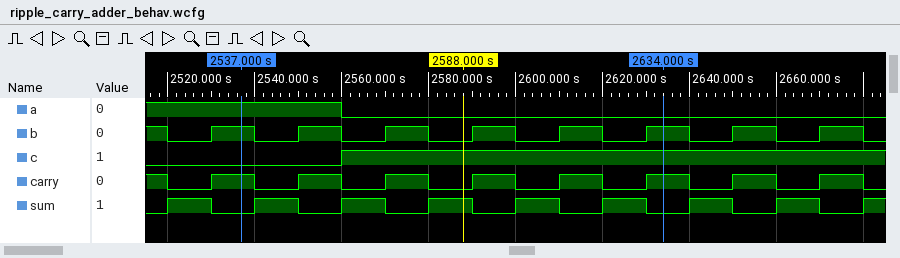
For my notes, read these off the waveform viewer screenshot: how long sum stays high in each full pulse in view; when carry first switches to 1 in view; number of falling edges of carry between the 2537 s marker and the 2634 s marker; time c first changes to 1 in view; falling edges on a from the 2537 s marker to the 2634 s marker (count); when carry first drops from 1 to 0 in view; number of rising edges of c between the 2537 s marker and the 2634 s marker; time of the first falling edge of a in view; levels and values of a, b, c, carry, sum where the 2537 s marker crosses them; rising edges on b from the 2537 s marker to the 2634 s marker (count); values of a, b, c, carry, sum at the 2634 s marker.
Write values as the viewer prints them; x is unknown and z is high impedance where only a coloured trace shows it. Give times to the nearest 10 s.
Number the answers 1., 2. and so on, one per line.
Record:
1. 10 s, 10 s, 10 s, 10 s, 10 s, 10 s, 10 s, 10 s
2. 2530 s
3. 5
4. 2560 s
5. 1
6. 2520 s
7. 1
8. 2560 s
9. a=1, b=1, c=0, carry=1, sum=0
10. 5
11. a=0, b=1, c=1, carry=1, sum=0
